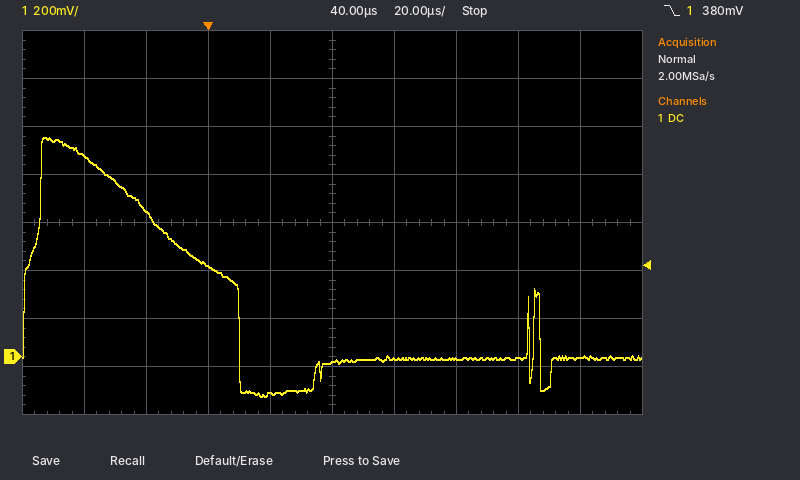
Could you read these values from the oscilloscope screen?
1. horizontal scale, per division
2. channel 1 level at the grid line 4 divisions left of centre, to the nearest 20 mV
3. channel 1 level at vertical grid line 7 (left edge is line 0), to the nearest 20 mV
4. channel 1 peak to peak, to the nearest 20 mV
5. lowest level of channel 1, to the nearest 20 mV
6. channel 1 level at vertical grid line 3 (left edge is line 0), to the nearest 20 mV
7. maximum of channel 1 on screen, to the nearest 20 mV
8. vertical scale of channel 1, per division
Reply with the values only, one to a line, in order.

20 µs
840 mV
0 mV
1.08 V
-160 mV
380 mV
920 mV
200 mV
